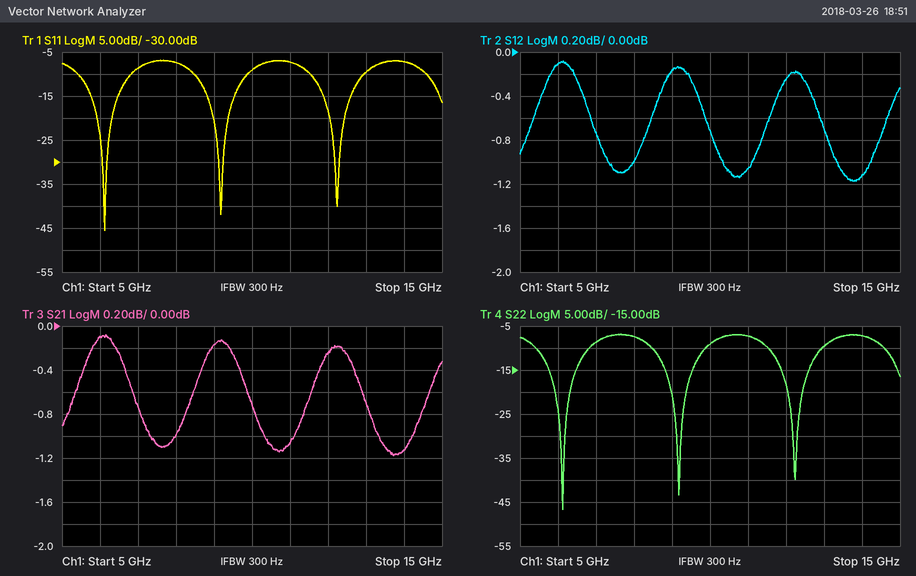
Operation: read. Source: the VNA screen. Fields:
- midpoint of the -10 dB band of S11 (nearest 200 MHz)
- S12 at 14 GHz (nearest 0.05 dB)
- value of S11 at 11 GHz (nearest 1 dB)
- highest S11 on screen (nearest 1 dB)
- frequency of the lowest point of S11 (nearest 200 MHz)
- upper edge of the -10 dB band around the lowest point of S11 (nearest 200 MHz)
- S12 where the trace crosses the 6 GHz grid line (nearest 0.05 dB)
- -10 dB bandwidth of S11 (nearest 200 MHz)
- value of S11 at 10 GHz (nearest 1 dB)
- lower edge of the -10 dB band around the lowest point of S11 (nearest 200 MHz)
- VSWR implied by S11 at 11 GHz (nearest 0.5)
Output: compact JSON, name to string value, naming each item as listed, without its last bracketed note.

{"midpoint of the -10 dB band of S11": "6.2 GHz", "S12 at 14 GHz": "-1.10 dB", "value of S11 at 11 GHz": "-7 dB", "highest S11 on screen": "-7 dB", "frequency of the lowest point of S11": "6.2 GHz", "upper edge of the -10 dB band around the lowest point of S11": "6.8 GHz", "S12 where the trace crosses the 6 GHz grid line": "-0.10 dB", "-10 dB bandwidth of S11": "1.4 GHz", "value of S11 at 10 GHz": "-9 dB", "lower edge of the -10 dB band around the lowest point of S11": "5.4 GHz", "VSWR implied by S11 at 11 GHz": "2.5"}
